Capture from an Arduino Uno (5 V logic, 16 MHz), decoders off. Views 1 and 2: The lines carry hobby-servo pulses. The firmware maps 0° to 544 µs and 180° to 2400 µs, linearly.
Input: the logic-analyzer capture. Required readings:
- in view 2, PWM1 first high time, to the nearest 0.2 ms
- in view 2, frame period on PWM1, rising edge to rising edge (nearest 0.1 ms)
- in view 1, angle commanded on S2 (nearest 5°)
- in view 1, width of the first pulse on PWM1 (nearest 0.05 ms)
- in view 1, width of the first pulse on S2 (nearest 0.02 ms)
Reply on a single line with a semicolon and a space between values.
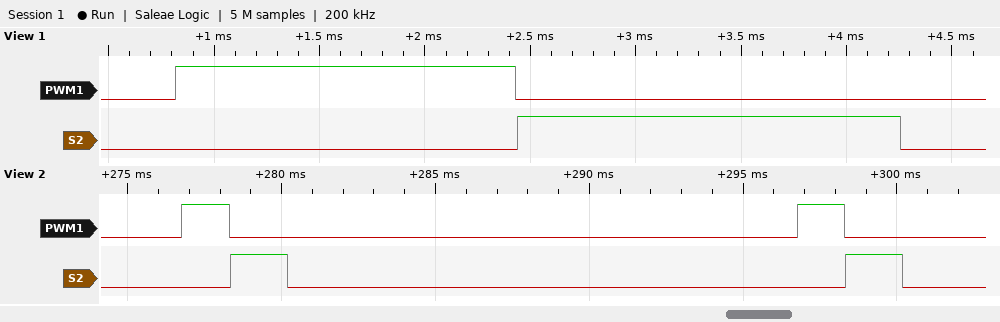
1.6 ms; 20.0 ms; 125°; 1.60 ms; 1.82 ms
